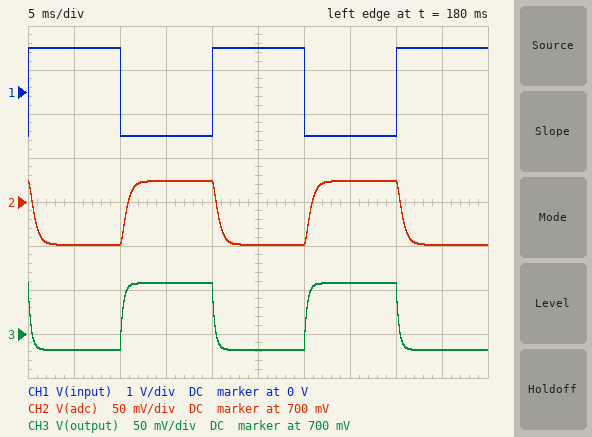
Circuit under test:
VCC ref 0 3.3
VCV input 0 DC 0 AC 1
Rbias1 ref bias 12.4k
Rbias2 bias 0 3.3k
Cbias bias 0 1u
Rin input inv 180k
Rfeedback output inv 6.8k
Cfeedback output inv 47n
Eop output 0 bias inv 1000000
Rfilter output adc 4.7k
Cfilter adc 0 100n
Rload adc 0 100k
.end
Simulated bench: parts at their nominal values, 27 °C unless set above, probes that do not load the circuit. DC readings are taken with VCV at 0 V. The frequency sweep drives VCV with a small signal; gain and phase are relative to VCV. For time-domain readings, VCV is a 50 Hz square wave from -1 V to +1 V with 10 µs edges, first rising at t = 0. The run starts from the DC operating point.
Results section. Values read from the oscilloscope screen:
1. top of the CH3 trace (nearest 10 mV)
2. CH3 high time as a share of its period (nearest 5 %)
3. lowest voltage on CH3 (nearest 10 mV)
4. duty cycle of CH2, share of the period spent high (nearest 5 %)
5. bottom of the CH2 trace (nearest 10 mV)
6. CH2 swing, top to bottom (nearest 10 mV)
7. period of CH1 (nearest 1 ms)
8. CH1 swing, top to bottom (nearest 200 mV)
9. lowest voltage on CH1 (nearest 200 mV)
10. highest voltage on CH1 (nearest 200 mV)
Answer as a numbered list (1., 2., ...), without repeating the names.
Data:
1. 760 mV
2. 50 %
3. 680 mV
4. 50 %
5. 650 mV
6. 70 mV
7. 20 ms
8. 2.0 V
9. -1.0 V
10. 1.0 V
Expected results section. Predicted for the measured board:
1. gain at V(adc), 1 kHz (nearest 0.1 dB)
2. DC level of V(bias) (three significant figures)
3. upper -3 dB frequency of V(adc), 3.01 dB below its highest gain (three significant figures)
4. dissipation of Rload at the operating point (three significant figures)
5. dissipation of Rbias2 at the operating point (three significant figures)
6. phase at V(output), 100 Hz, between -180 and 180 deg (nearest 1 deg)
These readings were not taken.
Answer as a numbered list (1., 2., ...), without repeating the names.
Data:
1. -45.4 dB
2. 694 mV
3. 265 Hz
4. 4.73 µW
5. 146 µW
6. 169 deg
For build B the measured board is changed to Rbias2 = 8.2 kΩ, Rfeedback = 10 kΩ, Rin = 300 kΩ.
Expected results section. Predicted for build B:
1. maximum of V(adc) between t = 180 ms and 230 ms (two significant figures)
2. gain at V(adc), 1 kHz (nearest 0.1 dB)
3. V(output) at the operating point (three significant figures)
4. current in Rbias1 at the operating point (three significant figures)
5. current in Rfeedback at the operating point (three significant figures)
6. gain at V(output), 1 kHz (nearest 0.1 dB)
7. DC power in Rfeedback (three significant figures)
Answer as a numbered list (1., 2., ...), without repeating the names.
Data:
1. 1.3 V
2. -49.3 dB
3. 1.36 V
4. 160 µA
5. 4.38 µA
6. -39.4 dB
7. 192 nW
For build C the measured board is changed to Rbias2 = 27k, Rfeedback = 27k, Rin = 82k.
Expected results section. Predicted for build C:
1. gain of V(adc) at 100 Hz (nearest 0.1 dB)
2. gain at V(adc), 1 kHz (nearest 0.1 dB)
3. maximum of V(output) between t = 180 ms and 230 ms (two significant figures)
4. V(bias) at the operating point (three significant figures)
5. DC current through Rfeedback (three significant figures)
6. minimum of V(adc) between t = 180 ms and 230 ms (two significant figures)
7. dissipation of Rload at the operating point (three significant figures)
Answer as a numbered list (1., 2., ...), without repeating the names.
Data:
1. -12.5 dB
2. -37.7 dB
3. 3.3 V
4. 2.26 V
5. 27.6 µA
6. 2.6 V
7. 82.4 µW
